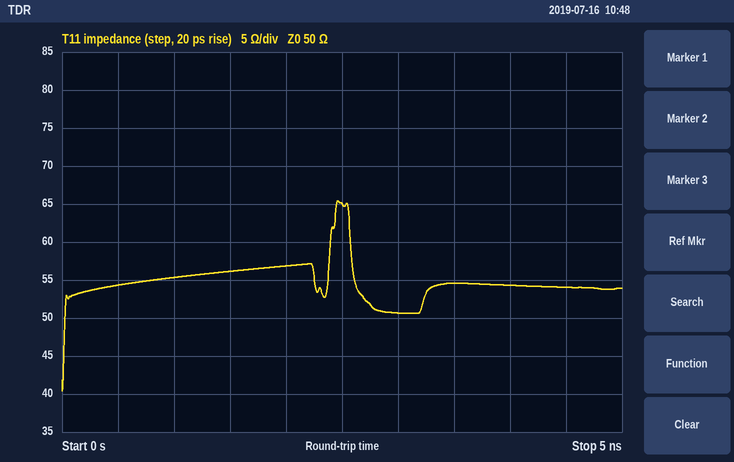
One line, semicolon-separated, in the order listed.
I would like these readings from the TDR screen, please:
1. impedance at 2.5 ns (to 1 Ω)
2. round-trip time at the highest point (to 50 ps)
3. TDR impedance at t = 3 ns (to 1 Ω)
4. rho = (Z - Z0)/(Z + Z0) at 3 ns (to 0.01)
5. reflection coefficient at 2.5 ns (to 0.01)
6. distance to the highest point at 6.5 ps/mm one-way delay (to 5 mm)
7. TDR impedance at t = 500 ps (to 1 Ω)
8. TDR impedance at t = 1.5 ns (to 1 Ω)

65 Ω; 2.45 ns; 51 Ω; +0.01; +0.13; 190 mm; 54 Ω; 56 Ω
